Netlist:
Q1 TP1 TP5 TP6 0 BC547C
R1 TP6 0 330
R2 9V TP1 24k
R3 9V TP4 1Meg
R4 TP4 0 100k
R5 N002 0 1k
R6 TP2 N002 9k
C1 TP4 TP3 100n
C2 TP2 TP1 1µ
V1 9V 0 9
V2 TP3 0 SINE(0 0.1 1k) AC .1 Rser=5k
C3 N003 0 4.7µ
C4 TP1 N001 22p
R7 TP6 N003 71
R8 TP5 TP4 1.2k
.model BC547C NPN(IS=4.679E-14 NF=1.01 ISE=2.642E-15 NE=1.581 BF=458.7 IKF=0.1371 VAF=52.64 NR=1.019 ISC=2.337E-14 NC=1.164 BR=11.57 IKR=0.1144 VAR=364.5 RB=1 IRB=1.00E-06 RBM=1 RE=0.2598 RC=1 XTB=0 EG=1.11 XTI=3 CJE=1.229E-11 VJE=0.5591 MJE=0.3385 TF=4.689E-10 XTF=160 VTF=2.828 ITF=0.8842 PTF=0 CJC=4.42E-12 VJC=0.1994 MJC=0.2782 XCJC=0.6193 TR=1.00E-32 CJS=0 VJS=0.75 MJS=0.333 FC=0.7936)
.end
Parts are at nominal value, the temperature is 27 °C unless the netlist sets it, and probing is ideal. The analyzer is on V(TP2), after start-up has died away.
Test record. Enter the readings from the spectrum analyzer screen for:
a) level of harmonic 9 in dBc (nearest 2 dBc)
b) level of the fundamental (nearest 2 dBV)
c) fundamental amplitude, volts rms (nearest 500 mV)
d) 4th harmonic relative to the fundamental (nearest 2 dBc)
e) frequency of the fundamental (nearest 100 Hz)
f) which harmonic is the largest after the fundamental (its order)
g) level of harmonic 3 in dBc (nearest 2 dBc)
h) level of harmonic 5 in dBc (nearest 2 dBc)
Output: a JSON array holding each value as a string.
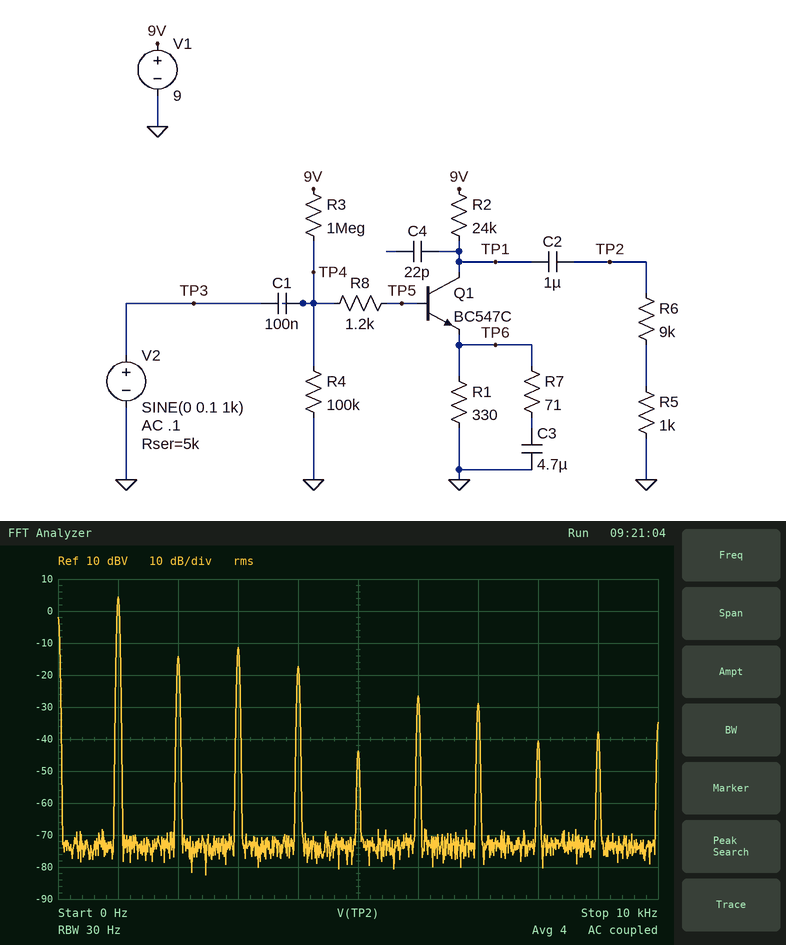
["-42 dBc", "4 dBV", "1.5 V", "-22 dBc", "1.0 kHz", "3", "-16 dBc", "-48 dBc"]
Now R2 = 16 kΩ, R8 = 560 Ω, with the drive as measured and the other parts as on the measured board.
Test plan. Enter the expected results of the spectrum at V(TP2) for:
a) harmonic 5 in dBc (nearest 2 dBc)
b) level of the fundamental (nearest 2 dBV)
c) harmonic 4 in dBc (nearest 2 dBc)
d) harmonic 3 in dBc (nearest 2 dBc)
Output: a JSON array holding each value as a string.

["-32 dBc", "6 dBV", "-24 dBc", "-20 dBc"]
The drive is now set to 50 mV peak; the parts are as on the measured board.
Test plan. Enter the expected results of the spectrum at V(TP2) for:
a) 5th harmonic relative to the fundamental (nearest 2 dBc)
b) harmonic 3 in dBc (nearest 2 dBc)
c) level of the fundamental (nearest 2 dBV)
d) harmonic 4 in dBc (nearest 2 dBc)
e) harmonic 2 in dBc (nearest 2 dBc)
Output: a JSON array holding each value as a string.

["-36 dBc", "-18 dBc", "0 dBV", "-30 dBc", "-24 dBc"]
